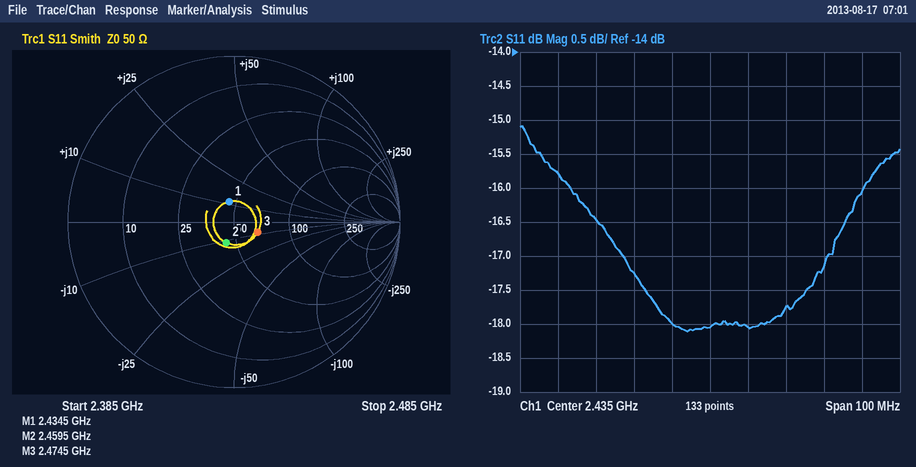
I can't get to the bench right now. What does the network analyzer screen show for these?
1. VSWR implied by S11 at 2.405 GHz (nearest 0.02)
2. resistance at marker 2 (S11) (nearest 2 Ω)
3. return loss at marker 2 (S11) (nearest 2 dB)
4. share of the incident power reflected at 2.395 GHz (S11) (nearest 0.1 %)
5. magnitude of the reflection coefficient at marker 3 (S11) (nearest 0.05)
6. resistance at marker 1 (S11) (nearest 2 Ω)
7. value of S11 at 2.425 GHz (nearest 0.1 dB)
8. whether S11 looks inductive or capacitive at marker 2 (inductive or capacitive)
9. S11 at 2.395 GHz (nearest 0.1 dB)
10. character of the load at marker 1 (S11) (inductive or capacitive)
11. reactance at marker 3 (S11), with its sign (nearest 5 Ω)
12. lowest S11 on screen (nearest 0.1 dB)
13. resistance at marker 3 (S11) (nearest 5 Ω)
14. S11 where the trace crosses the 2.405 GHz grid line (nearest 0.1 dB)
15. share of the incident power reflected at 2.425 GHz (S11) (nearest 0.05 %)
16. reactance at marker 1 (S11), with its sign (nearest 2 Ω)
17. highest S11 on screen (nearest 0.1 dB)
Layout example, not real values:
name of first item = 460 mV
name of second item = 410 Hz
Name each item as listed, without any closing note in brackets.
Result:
VSWR implied by S11 at 2.405 GHz = 1.36
resistance at marker 2 (S11) = 44 Ω
return loss at marker 2 (S11) = 18 dB
share of the incident power reflected at 2.395 GHz (S11) = 2.6 %
magnitude of the reflection coefficient at marker 3 (S11) = 0.15
resistance at marker 1 (S11) = 46 Ω
value of S11 at 2.425 GHz = -18.0 dB
whether S11 looks inductive or capacitive at marker 2 = capacitive
S11 at 2.395 GHz = -15.8 dB
character of the load at marker 1 (S11) = inductive
reactance at marker 3 (S11), with its sign = -10 Ω
lowest S11 on screen = -18.1 dB
resistance at marker 3 (S11) = 65 Ω
S11 where the trace crosses the 2.405 GHz grid line = -16.5 dB
share of the incident power reflected at 2.425 GHz (S11) = 1.60 %
reactance at marker 1 (S11), with its sign = +12 Ω
highest S11 on screen = -15.1 dB
